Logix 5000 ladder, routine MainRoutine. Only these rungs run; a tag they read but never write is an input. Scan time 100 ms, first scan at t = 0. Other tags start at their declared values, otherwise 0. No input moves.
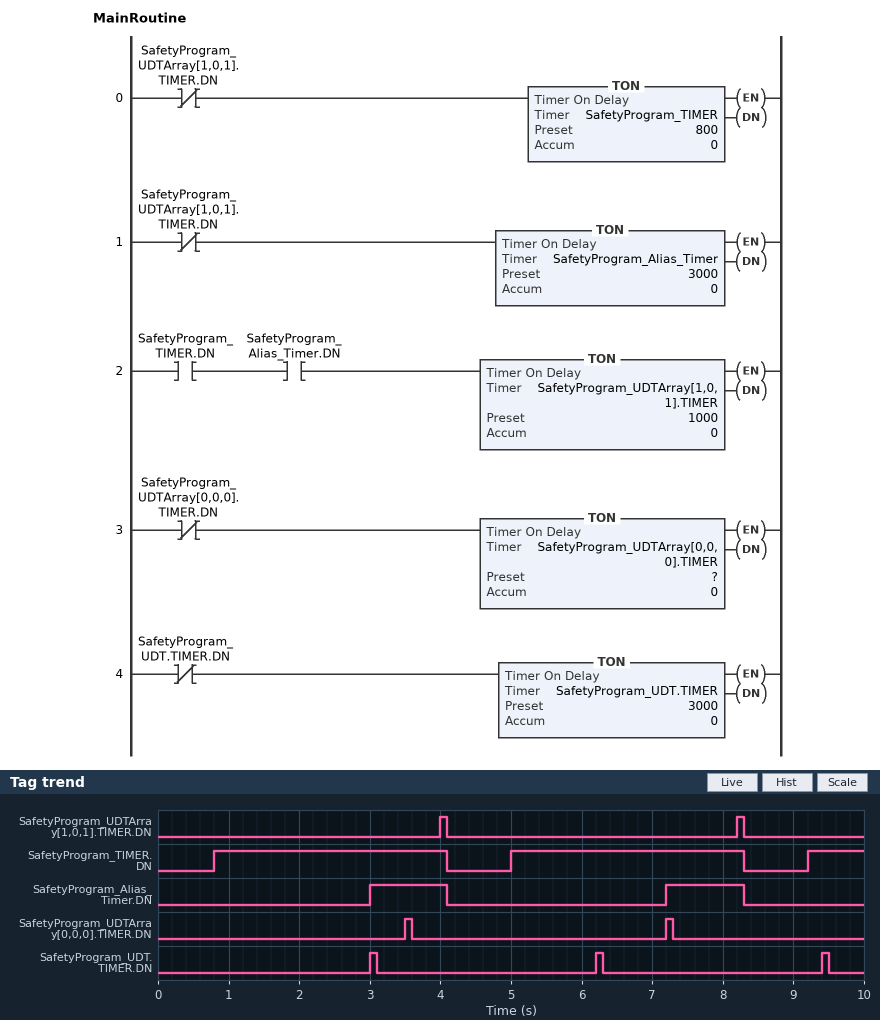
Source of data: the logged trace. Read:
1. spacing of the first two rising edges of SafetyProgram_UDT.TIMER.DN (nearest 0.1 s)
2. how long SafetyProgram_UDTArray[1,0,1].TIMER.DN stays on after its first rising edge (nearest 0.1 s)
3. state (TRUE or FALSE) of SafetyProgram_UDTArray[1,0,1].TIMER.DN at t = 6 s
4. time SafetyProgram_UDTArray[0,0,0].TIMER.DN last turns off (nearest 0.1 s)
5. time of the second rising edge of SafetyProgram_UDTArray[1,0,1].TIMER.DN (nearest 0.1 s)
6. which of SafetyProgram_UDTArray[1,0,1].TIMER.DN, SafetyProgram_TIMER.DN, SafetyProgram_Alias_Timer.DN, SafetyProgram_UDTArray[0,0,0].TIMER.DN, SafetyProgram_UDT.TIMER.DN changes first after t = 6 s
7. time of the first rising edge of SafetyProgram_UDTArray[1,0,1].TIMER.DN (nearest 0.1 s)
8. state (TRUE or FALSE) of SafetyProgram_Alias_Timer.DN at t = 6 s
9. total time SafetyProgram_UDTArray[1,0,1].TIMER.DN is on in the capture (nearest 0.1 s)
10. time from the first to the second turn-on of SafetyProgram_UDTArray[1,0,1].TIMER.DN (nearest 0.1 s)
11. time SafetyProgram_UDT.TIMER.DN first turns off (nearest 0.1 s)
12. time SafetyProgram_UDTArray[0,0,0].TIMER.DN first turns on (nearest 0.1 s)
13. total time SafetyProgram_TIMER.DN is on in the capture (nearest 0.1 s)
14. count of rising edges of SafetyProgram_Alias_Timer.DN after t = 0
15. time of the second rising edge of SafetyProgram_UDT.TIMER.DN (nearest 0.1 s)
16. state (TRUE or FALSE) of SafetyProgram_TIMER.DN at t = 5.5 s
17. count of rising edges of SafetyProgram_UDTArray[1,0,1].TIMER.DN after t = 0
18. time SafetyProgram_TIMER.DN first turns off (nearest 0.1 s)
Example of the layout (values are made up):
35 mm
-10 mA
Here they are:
3.2 s
0.1 s
FALSE
7.3 s
8.2 s
SafetyProgram_UDT.TIMER.DN
4.0 s
FALSE
0.2 s
4.2 s
3.1 s
3.5 s
7.4 s
2
6.2 s
TRUE
2
4.1 s
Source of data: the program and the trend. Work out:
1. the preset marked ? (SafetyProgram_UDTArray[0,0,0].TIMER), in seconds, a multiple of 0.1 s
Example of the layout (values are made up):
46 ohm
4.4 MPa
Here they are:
3.5 s
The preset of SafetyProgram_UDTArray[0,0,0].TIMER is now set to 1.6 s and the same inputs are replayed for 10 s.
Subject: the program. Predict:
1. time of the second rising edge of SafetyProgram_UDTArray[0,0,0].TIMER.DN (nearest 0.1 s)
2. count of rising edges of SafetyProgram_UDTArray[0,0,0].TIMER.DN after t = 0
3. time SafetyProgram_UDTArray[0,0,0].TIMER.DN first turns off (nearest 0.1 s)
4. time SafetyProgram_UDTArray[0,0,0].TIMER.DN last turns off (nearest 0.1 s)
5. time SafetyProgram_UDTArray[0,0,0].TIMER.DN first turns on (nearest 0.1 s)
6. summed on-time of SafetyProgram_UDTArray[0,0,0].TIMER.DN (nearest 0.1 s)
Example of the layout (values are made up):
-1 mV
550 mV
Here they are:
3.4 s
5
1.7 s
8.9 s
1.6 s
0.5 s
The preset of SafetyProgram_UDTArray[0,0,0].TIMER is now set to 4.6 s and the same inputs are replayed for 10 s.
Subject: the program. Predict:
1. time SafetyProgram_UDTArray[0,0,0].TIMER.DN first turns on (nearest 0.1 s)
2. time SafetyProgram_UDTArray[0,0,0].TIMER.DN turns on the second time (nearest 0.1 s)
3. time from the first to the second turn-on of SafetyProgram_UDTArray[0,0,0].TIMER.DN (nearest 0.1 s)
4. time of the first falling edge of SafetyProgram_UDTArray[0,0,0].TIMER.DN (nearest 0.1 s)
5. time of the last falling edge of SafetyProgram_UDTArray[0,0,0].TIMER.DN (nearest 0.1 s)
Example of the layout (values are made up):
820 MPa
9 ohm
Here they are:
4.6 s
9.4 s
4.8 s
4.7 s
9.5 s
